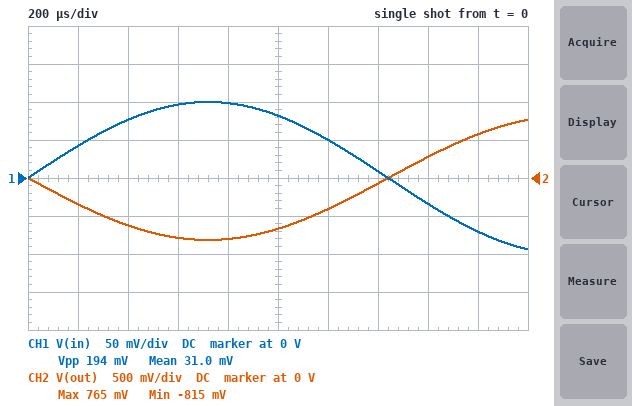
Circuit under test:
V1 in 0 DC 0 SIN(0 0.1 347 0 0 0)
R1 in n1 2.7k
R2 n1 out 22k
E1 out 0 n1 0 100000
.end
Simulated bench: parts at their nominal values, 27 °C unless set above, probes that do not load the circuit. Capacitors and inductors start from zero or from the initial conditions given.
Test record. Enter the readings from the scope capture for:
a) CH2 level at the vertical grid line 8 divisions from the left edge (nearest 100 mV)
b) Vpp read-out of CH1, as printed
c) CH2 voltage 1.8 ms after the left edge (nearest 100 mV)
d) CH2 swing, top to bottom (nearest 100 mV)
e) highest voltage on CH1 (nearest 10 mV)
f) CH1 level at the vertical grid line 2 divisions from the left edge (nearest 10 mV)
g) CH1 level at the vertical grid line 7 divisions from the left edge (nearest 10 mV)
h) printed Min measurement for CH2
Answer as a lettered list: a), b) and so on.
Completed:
a) 300 mV
b) 194 mV
c) 600 mV
d) 1.6 V
e) 100 mV
f) 80 mV
g) 10 mV
h) -815 mV
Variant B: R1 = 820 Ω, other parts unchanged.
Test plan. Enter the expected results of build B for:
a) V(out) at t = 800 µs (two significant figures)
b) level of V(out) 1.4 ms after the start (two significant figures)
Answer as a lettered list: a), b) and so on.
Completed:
a) -2.6 V
b) -240 mV
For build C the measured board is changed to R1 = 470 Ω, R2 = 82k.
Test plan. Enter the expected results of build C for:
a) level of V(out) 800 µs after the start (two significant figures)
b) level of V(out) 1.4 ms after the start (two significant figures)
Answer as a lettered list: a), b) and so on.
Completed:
a) -17 V
b) -1.6 V
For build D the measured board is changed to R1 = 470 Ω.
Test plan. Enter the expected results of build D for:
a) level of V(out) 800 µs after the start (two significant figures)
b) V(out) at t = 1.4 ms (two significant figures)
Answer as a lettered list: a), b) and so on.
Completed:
a) -4.6 V
b) -420 mV
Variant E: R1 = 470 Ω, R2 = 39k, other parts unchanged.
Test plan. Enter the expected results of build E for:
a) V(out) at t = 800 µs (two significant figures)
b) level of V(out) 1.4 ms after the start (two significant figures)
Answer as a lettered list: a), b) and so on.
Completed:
a) -8.2 V
b) -740 mV
